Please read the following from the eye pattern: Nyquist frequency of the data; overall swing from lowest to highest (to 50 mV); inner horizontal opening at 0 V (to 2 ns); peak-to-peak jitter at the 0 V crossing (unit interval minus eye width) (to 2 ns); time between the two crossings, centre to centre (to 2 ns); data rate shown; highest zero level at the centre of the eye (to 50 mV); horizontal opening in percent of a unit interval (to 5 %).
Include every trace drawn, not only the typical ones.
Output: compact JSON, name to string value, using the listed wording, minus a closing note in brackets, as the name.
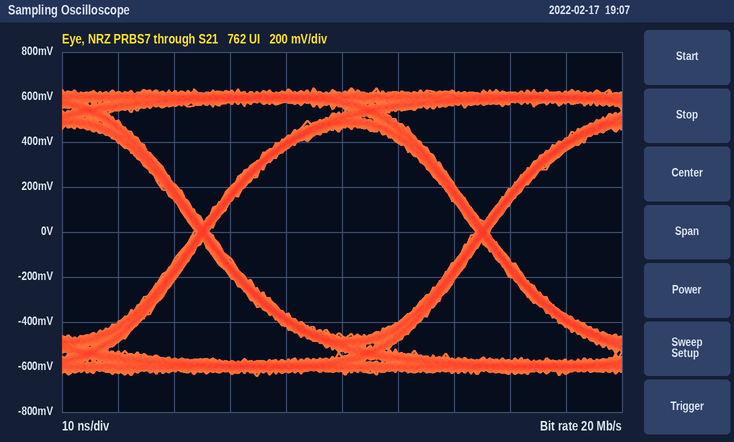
{"Nyquist frequency of the data": "10 MHz", "overall swing from lowest to highest": "1.30 V", "inner horizontal opening at 0 V": "48 ns", "peak-to-peak jitter at the 0 V crossing (unit interval minus eye width)": "2 ns", "time between the two crossings, centre to centre": "50 ns", "data rate shown": "20 Mb/s", "highest zero level at the centre of the eye": "-450 mV", "horizontal opening in percent of a unit interval": "95 %"}
